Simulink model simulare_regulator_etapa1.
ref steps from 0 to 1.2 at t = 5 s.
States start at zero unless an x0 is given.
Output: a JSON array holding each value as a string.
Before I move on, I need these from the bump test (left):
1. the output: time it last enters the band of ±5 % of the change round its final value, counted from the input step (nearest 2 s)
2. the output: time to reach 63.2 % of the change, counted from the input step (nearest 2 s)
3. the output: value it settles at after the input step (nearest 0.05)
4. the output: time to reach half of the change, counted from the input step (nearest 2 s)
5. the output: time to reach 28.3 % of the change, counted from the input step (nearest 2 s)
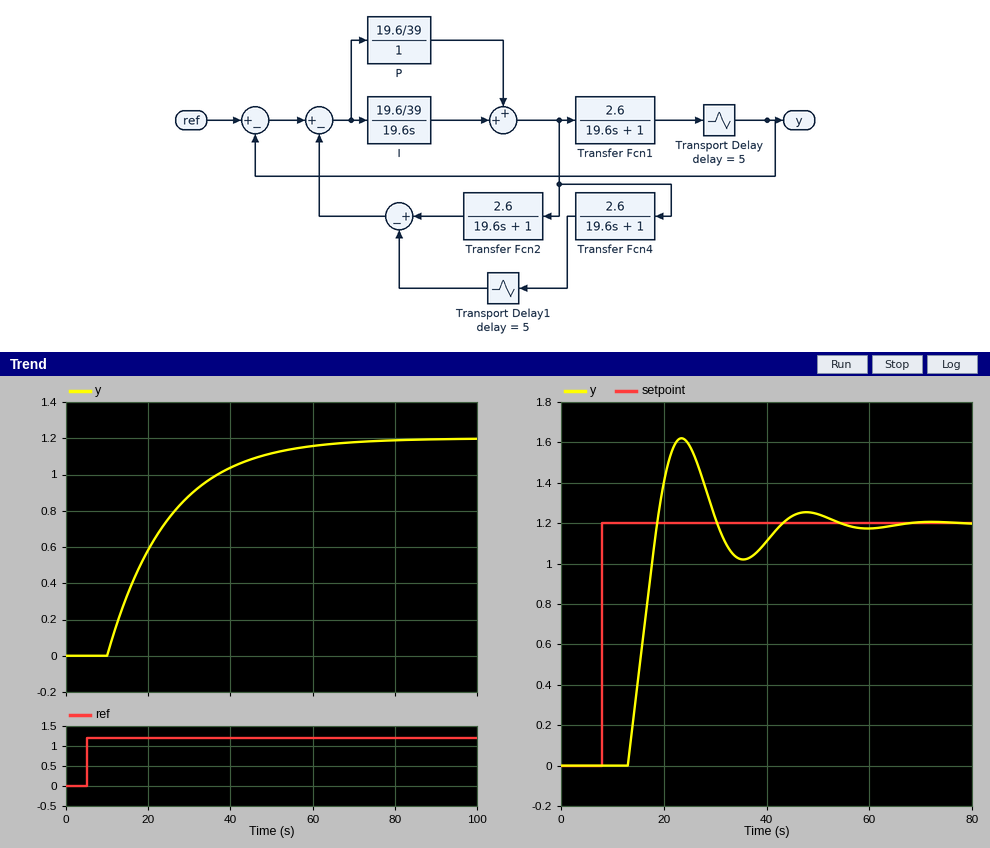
["50 s", "20 s", "1.20", "16 s", "10 s"]
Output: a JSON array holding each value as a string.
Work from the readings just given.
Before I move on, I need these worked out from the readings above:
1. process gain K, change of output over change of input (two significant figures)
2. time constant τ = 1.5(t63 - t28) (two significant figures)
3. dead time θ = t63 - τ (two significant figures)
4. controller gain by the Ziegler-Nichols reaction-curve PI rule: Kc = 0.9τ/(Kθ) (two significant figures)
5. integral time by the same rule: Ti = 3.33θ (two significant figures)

["1.0", "15 s", "5.0 s", "2.7", "17 s"]
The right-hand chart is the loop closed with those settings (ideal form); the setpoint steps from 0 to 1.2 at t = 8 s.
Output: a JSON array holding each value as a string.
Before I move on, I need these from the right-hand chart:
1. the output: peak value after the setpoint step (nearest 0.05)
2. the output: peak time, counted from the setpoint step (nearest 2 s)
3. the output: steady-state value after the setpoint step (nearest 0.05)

["1.60", "16 s", "1.20"]
